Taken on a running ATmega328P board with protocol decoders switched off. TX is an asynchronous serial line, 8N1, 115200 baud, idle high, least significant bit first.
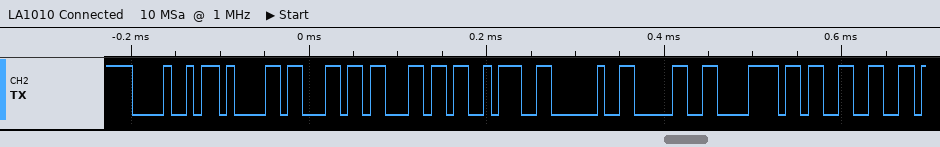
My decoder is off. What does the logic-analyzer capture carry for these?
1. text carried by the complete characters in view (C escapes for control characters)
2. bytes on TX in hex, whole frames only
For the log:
"Hall: 0x3"
0x48 0x61 0x6C 0x6C 0x3A 0x20 0x30 0x78 0x33
